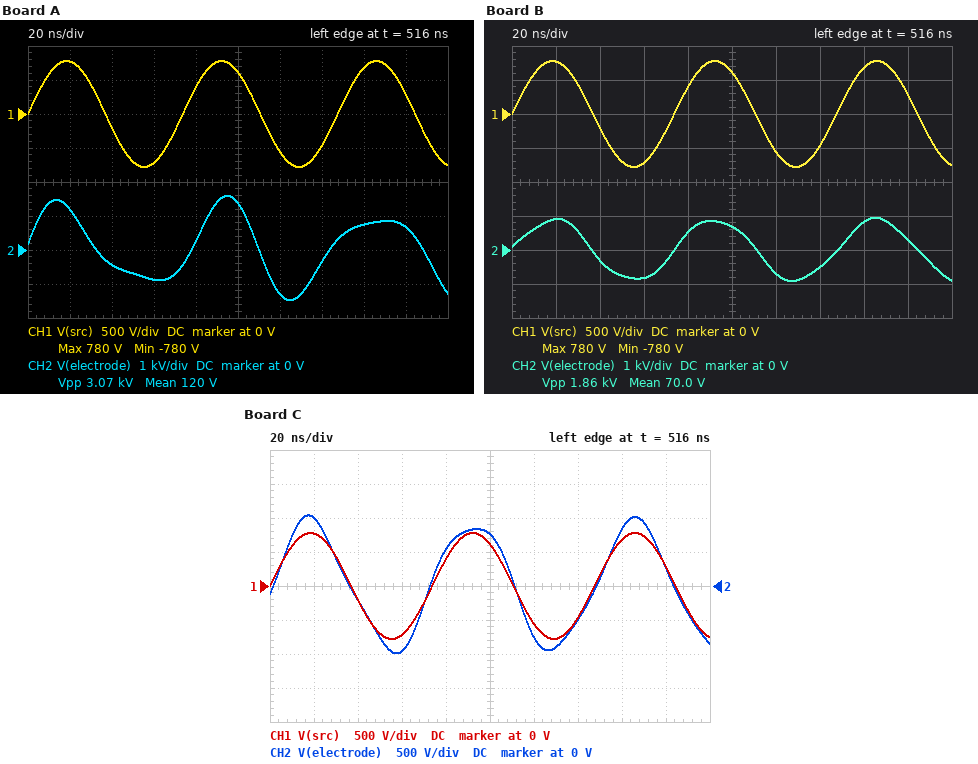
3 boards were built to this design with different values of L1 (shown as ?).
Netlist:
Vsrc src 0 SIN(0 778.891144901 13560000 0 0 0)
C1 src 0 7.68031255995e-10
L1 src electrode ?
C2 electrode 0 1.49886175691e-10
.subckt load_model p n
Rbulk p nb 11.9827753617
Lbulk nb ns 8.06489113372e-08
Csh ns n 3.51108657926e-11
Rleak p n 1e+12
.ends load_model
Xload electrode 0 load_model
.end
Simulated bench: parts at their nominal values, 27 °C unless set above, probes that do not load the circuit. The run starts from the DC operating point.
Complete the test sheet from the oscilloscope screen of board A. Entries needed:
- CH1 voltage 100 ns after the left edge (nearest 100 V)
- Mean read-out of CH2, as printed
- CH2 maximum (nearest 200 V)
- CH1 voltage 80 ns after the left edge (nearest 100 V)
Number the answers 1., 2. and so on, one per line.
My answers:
1. 600 V
2. 120 V
3. 1.6 kV
4. 400 V
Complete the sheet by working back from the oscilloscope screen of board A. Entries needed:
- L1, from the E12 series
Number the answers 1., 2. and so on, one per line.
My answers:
1. 270 nH
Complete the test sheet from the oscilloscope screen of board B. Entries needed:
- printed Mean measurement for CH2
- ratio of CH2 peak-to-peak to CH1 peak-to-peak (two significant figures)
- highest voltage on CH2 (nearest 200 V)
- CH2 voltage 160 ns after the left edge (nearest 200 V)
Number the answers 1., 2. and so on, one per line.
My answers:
1. 70.0 V
2. 1.2
3. 1.0 kV
4. 800 V
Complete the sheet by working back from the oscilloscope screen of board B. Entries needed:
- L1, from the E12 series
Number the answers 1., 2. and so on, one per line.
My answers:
1. 100 nH
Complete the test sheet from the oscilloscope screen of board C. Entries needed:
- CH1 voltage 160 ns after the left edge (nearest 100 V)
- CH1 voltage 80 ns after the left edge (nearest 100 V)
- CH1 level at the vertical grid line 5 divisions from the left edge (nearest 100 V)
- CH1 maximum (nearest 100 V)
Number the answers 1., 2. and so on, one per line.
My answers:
1. 700 V
2. 400 V
3. 600 V
4. 800 V
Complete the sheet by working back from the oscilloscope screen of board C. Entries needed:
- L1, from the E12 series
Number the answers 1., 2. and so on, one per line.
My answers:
1. 120 nH
